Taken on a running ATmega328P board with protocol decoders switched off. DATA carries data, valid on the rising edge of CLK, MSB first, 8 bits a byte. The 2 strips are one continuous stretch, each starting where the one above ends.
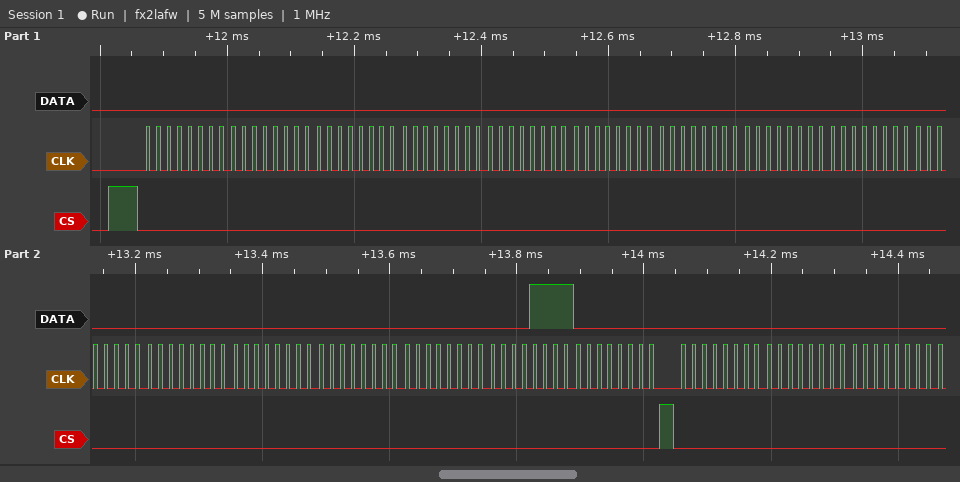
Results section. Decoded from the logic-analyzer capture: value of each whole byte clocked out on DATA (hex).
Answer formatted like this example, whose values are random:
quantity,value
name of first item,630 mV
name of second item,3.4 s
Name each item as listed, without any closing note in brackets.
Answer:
quantity,value
value of each whole byte clocked out on DATA,00 00 00 00 00 00 00 00 00 00 00 00 00 00 0F 00 00 00 00
